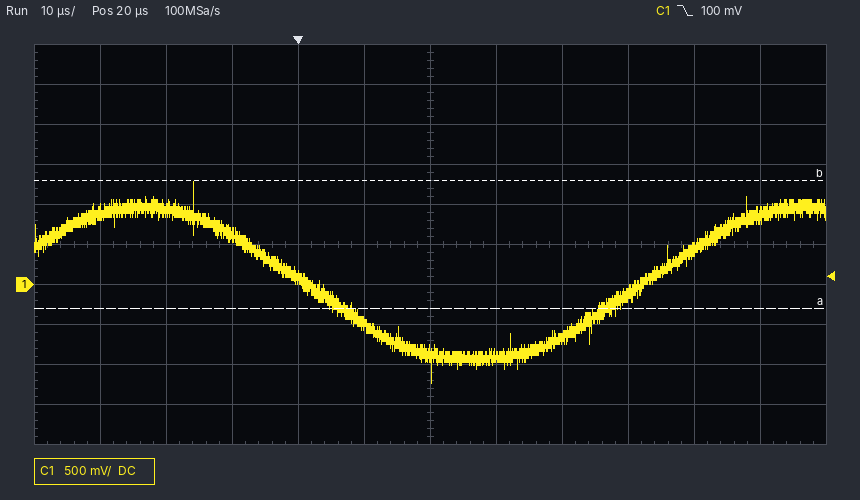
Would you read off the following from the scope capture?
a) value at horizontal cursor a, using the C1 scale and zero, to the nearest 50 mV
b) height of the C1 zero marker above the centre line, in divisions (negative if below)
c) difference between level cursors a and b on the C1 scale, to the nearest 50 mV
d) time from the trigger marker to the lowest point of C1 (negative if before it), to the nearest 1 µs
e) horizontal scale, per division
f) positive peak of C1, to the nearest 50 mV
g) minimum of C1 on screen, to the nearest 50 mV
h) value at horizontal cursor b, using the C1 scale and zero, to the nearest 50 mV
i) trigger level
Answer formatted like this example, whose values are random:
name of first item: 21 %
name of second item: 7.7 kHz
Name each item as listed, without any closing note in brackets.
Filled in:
value at horizontal cursor a, using the C1 scale and zero, to the nearest 50 mV: -300 mV
height of the C1 zero marker above the centre line, in divisions: -1.0 div
difference between level cursors a and b on the C1 scale, to the nearest 50 mV: 1.60 V
time from the trigger marker to the lowest point of C1 (negative if before it), to the nearest 1 µs: +20 µs
horizontal scale, per division: 10 µs
positive peak of C1, to the nearest 50 mV: 1.30 V
minimum of C1 on screen, to the nearest 50 mV: -1.25 V
value at horizontal cursor b, using the C1 scale and zero, to the nearest 50 mV: 1.30 V
trigger level: 100 mV
